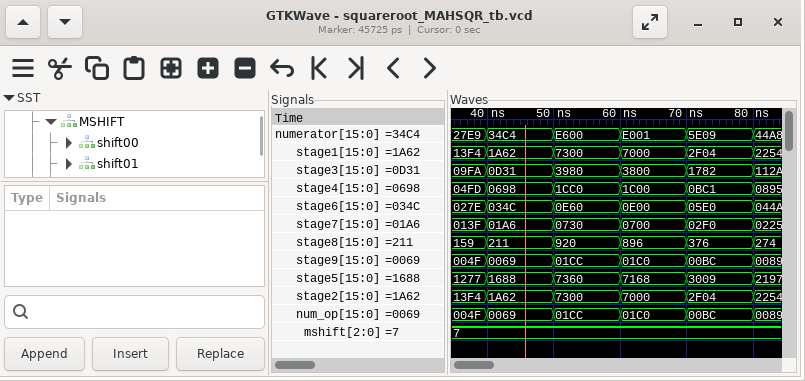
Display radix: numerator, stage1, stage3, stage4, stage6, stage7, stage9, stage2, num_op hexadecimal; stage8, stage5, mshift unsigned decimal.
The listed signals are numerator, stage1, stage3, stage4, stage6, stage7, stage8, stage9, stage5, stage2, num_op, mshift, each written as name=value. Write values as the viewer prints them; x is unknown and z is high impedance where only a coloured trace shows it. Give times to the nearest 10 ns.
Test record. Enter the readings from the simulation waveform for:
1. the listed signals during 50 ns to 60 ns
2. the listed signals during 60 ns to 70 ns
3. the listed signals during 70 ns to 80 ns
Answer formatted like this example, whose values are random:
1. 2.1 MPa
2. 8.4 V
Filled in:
1. numerator=E600, stage1=7300, stage3=3980, stage4=1CC0, stage6=0E60, stage7=0730, stage8=920, stage9=01CC, stage5=7360, stage2=7300, num_op=01CC, mshift=7
2. numerator=E001, stage1=7000, stage3=3800, stage4=1C00, stage6=0E00, stage7=0700, stage8=896, stage9=01C0, stage5=7168, stage2=7000, num_op=01C0, mshift=7
3. numerator=5E09, stage1=2F04, stage3=1782, stage4=0BC1, stage6=05E0, stage7=02F0, stage8=376, stage9=00BC, stage5=3009, stage2=2F04, num_op=00BC, mshift=7
